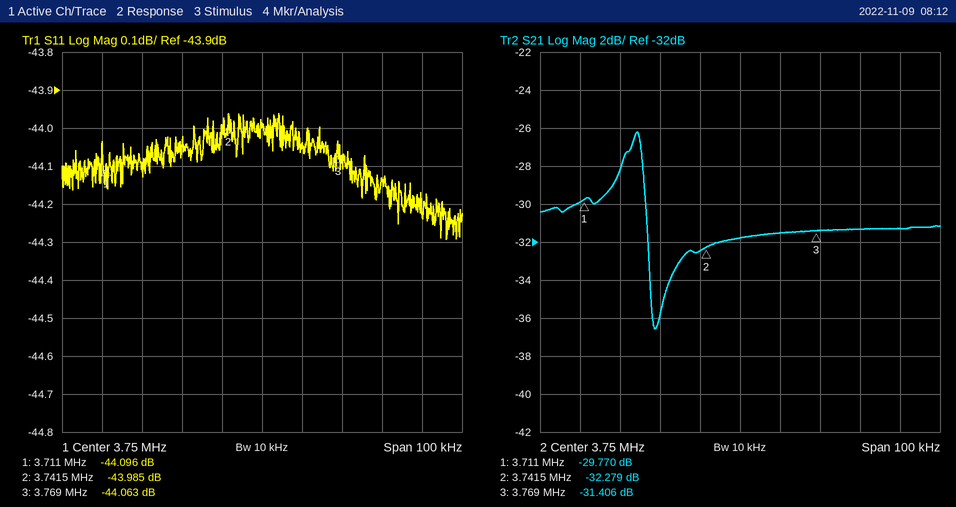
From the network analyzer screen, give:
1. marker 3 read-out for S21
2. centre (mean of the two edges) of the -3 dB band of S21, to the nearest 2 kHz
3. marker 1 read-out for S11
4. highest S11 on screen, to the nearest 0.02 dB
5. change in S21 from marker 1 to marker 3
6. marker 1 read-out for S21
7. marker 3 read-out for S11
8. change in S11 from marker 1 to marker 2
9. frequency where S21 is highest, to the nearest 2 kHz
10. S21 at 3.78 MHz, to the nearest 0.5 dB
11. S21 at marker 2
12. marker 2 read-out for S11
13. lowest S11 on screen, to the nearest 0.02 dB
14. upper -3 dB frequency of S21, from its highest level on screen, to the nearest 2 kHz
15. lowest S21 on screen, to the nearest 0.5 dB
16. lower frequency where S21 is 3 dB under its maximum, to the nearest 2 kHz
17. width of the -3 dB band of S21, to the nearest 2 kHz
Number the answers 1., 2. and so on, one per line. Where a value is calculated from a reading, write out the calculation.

1. -31.406 dB
2. 3.722 MHz
3. -44.096 dB
4. -43.96 dB
5. -31.406 − (-29.77) = -1.636 dB
6. -29.770 dB
7. -44.063 dB
8. -43.985 − (-44.096) = 0.111 dB
9. 3.724 MHz
10. -31.5 dB
11. -32.279 dB
12. -43.985 dB
13. -44.30 dB
14. 3.726 MHz
15. -36.5 dB
16. 3.718 MHz
17. 3.726 MHz − 3.718 MHz = 8 kHz
